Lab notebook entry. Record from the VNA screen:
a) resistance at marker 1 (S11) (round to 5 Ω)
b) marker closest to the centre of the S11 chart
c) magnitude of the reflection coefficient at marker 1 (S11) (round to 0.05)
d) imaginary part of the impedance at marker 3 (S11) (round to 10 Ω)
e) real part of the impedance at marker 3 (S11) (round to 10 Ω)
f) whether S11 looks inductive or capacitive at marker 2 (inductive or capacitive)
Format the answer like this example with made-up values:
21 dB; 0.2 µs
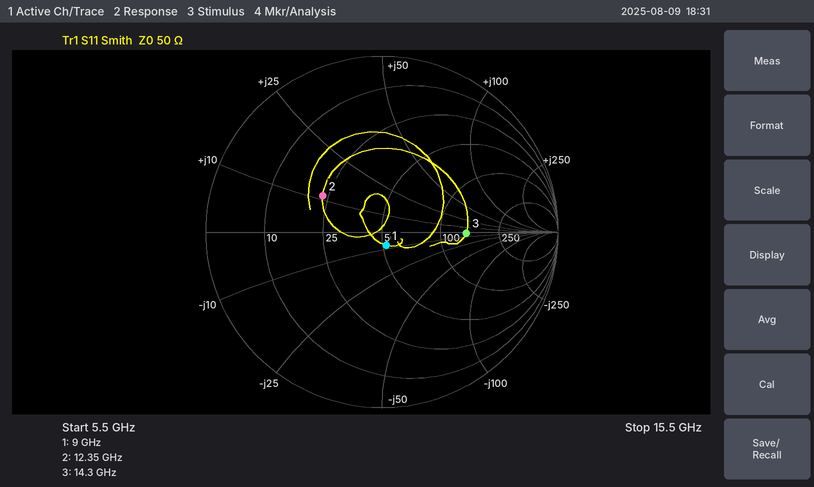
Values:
50 Ω; marker 1; 0.10; 0 Ω; 140 Ω; inductive
